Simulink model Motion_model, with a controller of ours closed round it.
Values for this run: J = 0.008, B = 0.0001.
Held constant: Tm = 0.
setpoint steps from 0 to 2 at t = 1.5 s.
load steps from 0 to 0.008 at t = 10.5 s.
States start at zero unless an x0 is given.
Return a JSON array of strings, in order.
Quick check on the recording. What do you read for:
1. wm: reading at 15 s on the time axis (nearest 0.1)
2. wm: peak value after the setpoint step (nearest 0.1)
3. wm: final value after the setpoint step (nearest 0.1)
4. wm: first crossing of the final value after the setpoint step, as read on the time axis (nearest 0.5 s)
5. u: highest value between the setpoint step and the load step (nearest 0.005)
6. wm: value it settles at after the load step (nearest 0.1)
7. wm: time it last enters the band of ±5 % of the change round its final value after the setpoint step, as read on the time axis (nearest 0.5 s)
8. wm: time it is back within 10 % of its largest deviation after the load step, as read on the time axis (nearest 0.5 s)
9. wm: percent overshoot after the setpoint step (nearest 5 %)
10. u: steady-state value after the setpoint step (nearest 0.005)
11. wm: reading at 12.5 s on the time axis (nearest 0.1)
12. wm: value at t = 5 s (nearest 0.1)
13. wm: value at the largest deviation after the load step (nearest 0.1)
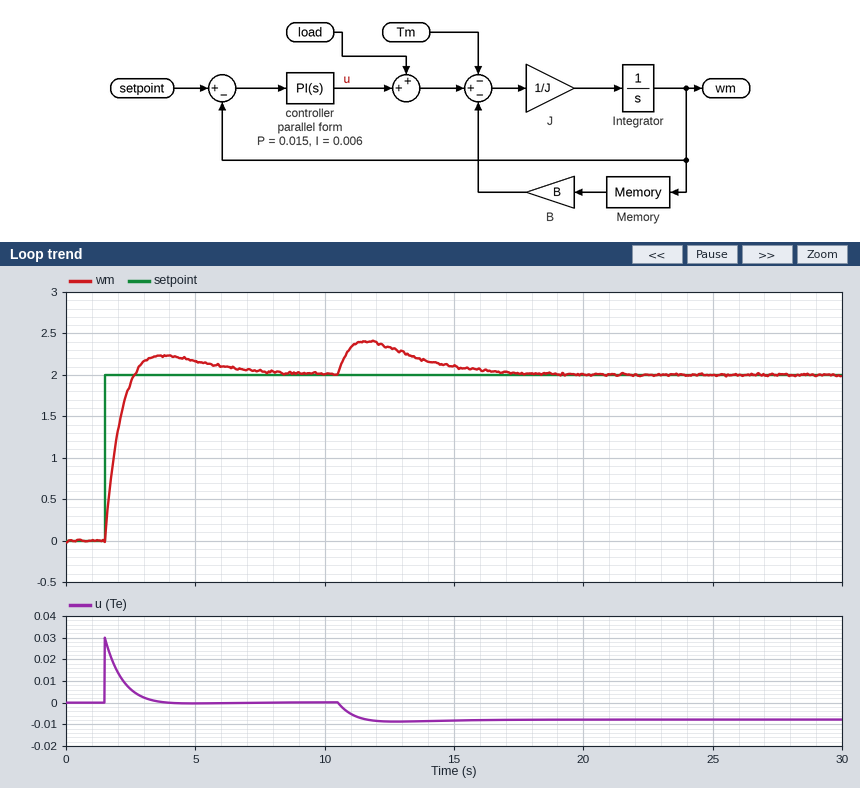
["2.1", "2.2", "2.0", "2.5 s", "0.030", "2.0", "6.0 s", "16.5 s", "10 %", "0.000", "2.3", "2.2", "2.4"]
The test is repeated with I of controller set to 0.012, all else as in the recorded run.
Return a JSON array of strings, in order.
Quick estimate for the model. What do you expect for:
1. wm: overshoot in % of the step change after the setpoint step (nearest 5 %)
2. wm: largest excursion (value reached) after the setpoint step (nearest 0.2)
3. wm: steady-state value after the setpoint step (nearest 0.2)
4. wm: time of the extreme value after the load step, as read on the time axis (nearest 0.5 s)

["20 %", "2.4", "2.0", "11.5 s"]
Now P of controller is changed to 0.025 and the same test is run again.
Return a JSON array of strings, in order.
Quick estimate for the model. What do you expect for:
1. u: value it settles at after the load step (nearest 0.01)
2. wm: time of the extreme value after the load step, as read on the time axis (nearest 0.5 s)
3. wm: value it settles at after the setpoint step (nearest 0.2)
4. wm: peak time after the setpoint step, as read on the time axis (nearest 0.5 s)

["-0.01", "11.5 s", "2.0", "3.5 s"]
